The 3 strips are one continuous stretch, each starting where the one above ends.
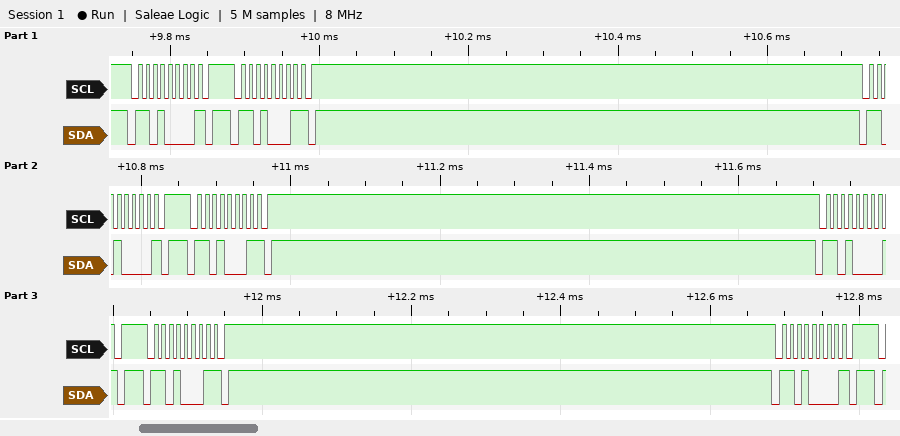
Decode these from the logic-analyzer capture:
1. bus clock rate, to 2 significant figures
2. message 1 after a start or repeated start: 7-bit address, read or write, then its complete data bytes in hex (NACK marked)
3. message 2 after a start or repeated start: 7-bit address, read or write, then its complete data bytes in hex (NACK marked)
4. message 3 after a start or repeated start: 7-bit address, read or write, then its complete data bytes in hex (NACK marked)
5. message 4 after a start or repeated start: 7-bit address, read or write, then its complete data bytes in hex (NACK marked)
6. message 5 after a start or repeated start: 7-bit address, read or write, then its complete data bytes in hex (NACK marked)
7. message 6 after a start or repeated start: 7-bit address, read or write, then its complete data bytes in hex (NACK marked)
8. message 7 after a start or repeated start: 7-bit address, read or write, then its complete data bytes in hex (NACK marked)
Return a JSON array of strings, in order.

["100 kHz", "0x68 write NACK", "0x68 read NACK", "0x68 write NACK", "0x68 read NACK", "0x68 write NACK", "0x68 read NACK", "0x68 write NACK"]
